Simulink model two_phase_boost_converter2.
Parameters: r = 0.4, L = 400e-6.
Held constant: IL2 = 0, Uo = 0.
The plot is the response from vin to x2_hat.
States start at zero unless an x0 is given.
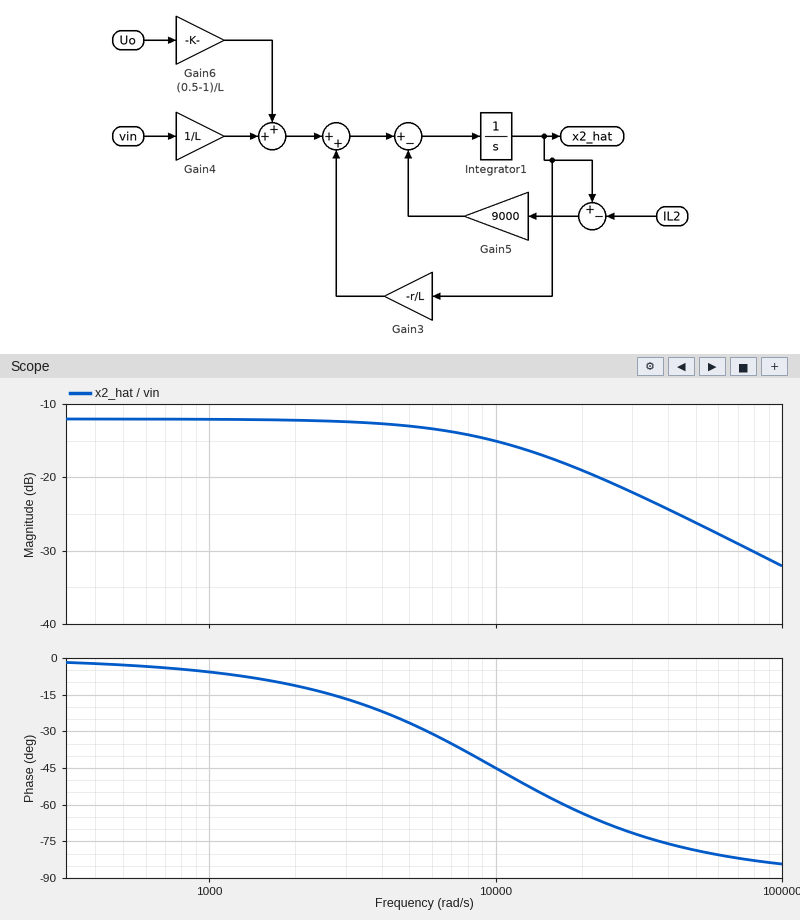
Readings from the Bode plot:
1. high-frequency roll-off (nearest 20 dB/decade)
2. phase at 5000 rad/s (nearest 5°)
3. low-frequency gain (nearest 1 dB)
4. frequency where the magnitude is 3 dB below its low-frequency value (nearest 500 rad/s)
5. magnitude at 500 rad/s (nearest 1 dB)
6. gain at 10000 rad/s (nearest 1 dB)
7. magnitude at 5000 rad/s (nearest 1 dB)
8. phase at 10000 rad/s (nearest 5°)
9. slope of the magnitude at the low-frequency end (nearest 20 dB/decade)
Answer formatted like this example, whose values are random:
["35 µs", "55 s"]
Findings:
["-20 dB/decade", "-25°", "-12 dB", "10000 rad/s", "-12 dB", "-15 dB", "-13 dB", "-45°", "0 dB/decade"]
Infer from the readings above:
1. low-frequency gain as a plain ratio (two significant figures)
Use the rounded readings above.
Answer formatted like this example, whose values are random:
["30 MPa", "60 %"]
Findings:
["0.25"]
